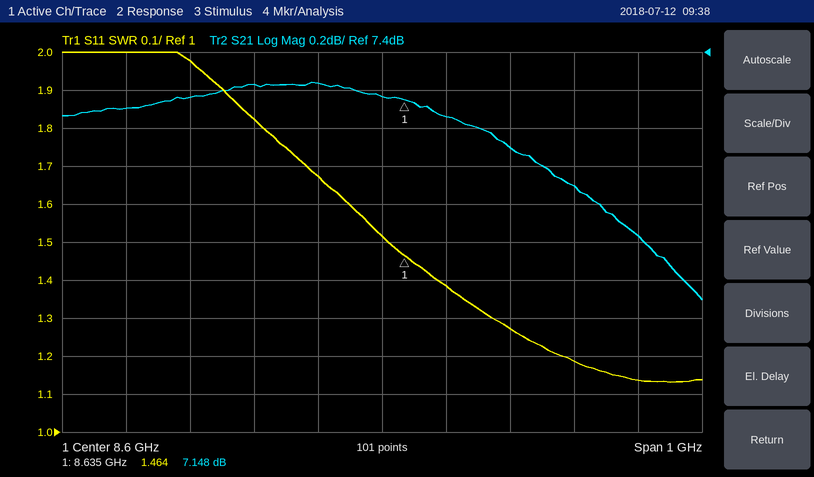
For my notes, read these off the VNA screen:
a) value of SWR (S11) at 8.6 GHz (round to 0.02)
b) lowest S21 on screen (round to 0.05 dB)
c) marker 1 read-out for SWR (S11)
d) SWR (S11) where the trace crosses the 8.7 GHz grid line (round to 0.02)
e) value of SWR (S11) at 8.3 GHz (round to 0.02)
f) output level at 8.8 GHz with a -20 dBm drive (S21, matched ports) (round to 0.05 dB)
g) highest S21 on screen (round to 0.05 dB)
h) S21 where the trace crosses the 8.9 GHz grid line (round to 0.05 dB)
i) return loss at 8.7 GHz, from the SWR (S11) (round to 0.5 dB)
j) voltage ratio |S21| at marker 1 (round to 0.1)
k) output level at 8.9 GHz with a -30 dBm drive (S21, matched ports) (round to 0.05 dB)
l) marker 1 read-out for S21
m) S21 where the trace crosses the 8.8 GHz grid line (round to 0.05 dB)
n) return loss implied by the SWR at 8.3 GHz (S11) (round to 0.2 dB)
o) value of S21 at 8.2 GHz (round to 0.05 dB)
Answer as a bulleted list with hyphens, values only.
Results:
- 1.52
- 6.10 dB
- 1.464
- 1.38
- 1.98
- -13.10 dBm
- 7.25 dB
- 6.70 dB
- 16.0 dB
- 2.3
- -23.30 dBm
- 7.148 dB
- 6.90 dB
- 9.6 dB
- 7.10 dB
